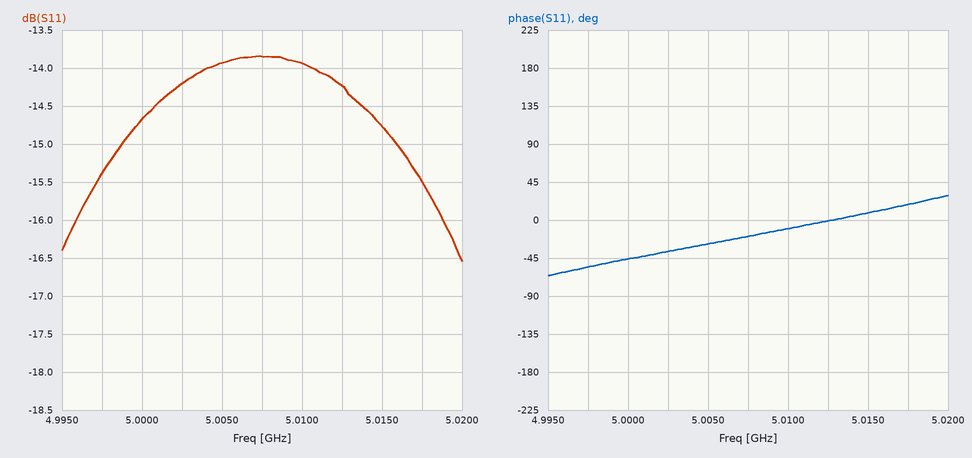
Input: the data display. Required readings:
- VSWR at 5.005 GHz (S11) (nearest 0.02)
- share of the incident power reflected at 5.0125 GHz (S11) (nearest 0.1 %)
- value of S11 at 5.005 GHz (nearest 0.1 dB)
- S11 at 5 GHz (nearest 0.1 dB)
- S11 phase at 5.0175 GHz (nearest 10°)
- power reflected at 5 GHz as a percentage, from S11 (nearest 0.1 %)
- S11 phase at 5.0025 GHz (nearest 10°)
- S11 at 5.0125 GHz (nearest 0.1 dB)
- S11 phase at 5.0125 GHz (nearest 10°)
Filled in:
1.50
3.8 %
-13.9 dB
-14.7 dB
20°
3.4 %
-40°
-14.2 dB
0°
